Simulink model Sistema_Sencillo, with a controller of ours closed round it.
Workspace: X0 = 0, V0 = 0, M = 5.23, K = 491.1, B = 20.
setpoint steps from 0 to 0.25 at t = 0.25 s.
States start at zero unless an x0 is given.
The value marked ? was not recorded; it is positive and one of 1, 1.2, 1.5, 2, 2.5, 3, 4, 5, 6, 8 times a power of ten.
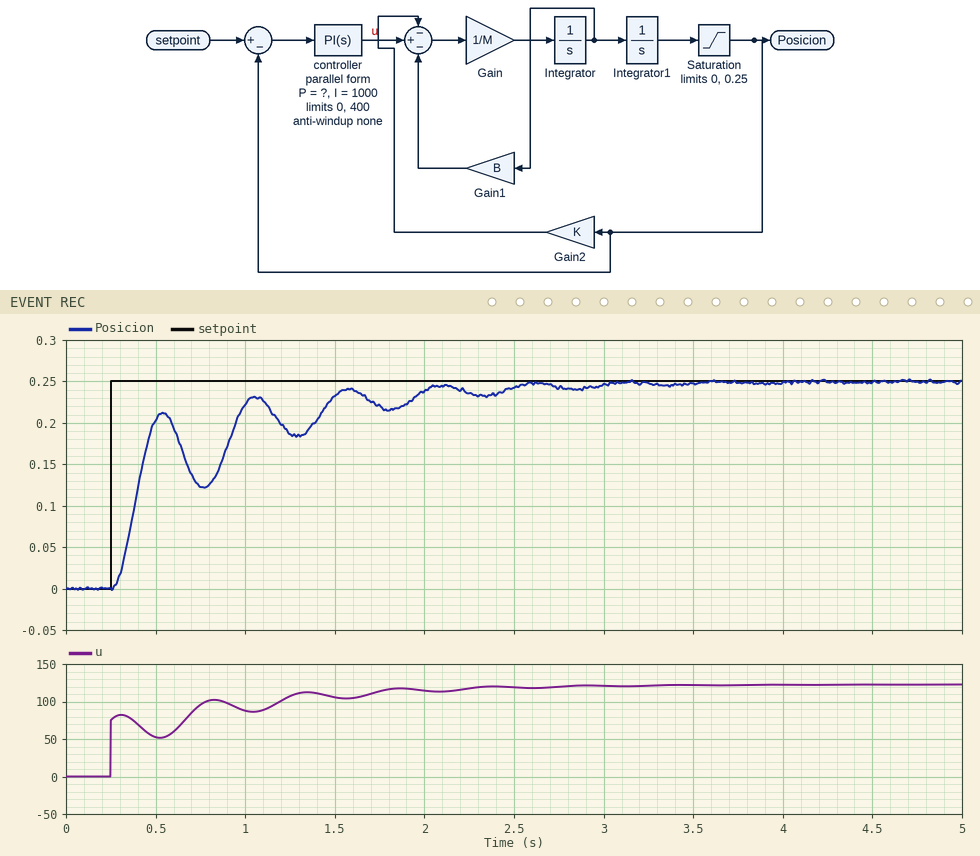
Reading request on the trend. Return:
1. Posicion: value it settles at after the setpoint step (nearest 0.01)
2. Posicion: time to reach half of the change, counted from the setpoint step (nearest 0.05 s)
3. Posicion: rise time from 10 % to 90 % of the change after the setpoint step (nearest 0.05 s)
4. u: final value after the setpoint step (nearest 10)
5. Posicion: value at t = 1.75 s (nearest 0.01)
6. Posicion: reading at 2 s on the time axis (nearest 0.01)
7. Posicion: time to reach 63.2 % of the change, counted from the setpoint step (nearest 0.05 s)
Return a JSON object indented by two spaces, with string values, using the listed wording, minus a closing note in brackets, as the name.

{
  "Posicion: value it settles at after the setpoint step": "0.25",
  "Posicion: time to reach half of the change, counted from the setpoint step": "0.15 s",
  "Posicion: rise time from 10 % to 90 % of the change after the setpoint step": "0.70 s",
  "u: final value after the setpoint step": "120",
  "Posicion: value at t = 1.75 s": "0.22",
  "Posicion: reading at 2 s on the time axis": "0.24",
  "Posicion: time to reach 63.2 % of the change, counted from the setpoint step": "0.20 s"
}
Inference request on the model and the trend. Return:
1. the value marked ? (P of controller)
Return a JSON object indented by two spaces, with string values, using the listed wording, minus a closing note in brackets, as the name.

{
  "the value marked ?": "300"
}
